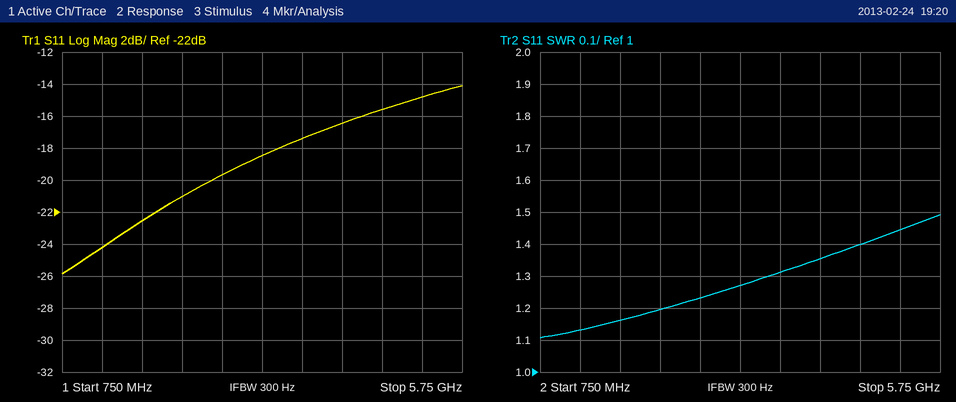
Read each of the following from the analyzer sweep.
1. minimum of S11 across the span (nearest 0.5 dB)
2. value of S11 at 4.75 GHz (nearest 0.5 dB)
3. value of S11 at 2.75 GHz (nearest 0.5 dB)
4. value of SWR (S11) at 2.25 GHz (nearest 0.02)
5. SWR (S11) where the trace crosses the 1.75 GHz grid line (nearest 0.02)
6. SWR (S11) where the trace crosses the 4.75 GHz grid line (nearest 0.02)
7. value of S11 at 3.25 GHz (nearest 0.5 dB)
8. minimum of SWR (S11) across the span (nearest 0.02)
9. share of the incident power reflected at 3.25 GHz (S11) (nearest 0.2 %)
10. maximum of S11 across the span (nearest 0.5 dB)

-26.0 dB
-15.5 dB
-19.5 dB
1.20
1.16
1.40
-18.5 dB
1.10
1.4 %
-14.0 dB
